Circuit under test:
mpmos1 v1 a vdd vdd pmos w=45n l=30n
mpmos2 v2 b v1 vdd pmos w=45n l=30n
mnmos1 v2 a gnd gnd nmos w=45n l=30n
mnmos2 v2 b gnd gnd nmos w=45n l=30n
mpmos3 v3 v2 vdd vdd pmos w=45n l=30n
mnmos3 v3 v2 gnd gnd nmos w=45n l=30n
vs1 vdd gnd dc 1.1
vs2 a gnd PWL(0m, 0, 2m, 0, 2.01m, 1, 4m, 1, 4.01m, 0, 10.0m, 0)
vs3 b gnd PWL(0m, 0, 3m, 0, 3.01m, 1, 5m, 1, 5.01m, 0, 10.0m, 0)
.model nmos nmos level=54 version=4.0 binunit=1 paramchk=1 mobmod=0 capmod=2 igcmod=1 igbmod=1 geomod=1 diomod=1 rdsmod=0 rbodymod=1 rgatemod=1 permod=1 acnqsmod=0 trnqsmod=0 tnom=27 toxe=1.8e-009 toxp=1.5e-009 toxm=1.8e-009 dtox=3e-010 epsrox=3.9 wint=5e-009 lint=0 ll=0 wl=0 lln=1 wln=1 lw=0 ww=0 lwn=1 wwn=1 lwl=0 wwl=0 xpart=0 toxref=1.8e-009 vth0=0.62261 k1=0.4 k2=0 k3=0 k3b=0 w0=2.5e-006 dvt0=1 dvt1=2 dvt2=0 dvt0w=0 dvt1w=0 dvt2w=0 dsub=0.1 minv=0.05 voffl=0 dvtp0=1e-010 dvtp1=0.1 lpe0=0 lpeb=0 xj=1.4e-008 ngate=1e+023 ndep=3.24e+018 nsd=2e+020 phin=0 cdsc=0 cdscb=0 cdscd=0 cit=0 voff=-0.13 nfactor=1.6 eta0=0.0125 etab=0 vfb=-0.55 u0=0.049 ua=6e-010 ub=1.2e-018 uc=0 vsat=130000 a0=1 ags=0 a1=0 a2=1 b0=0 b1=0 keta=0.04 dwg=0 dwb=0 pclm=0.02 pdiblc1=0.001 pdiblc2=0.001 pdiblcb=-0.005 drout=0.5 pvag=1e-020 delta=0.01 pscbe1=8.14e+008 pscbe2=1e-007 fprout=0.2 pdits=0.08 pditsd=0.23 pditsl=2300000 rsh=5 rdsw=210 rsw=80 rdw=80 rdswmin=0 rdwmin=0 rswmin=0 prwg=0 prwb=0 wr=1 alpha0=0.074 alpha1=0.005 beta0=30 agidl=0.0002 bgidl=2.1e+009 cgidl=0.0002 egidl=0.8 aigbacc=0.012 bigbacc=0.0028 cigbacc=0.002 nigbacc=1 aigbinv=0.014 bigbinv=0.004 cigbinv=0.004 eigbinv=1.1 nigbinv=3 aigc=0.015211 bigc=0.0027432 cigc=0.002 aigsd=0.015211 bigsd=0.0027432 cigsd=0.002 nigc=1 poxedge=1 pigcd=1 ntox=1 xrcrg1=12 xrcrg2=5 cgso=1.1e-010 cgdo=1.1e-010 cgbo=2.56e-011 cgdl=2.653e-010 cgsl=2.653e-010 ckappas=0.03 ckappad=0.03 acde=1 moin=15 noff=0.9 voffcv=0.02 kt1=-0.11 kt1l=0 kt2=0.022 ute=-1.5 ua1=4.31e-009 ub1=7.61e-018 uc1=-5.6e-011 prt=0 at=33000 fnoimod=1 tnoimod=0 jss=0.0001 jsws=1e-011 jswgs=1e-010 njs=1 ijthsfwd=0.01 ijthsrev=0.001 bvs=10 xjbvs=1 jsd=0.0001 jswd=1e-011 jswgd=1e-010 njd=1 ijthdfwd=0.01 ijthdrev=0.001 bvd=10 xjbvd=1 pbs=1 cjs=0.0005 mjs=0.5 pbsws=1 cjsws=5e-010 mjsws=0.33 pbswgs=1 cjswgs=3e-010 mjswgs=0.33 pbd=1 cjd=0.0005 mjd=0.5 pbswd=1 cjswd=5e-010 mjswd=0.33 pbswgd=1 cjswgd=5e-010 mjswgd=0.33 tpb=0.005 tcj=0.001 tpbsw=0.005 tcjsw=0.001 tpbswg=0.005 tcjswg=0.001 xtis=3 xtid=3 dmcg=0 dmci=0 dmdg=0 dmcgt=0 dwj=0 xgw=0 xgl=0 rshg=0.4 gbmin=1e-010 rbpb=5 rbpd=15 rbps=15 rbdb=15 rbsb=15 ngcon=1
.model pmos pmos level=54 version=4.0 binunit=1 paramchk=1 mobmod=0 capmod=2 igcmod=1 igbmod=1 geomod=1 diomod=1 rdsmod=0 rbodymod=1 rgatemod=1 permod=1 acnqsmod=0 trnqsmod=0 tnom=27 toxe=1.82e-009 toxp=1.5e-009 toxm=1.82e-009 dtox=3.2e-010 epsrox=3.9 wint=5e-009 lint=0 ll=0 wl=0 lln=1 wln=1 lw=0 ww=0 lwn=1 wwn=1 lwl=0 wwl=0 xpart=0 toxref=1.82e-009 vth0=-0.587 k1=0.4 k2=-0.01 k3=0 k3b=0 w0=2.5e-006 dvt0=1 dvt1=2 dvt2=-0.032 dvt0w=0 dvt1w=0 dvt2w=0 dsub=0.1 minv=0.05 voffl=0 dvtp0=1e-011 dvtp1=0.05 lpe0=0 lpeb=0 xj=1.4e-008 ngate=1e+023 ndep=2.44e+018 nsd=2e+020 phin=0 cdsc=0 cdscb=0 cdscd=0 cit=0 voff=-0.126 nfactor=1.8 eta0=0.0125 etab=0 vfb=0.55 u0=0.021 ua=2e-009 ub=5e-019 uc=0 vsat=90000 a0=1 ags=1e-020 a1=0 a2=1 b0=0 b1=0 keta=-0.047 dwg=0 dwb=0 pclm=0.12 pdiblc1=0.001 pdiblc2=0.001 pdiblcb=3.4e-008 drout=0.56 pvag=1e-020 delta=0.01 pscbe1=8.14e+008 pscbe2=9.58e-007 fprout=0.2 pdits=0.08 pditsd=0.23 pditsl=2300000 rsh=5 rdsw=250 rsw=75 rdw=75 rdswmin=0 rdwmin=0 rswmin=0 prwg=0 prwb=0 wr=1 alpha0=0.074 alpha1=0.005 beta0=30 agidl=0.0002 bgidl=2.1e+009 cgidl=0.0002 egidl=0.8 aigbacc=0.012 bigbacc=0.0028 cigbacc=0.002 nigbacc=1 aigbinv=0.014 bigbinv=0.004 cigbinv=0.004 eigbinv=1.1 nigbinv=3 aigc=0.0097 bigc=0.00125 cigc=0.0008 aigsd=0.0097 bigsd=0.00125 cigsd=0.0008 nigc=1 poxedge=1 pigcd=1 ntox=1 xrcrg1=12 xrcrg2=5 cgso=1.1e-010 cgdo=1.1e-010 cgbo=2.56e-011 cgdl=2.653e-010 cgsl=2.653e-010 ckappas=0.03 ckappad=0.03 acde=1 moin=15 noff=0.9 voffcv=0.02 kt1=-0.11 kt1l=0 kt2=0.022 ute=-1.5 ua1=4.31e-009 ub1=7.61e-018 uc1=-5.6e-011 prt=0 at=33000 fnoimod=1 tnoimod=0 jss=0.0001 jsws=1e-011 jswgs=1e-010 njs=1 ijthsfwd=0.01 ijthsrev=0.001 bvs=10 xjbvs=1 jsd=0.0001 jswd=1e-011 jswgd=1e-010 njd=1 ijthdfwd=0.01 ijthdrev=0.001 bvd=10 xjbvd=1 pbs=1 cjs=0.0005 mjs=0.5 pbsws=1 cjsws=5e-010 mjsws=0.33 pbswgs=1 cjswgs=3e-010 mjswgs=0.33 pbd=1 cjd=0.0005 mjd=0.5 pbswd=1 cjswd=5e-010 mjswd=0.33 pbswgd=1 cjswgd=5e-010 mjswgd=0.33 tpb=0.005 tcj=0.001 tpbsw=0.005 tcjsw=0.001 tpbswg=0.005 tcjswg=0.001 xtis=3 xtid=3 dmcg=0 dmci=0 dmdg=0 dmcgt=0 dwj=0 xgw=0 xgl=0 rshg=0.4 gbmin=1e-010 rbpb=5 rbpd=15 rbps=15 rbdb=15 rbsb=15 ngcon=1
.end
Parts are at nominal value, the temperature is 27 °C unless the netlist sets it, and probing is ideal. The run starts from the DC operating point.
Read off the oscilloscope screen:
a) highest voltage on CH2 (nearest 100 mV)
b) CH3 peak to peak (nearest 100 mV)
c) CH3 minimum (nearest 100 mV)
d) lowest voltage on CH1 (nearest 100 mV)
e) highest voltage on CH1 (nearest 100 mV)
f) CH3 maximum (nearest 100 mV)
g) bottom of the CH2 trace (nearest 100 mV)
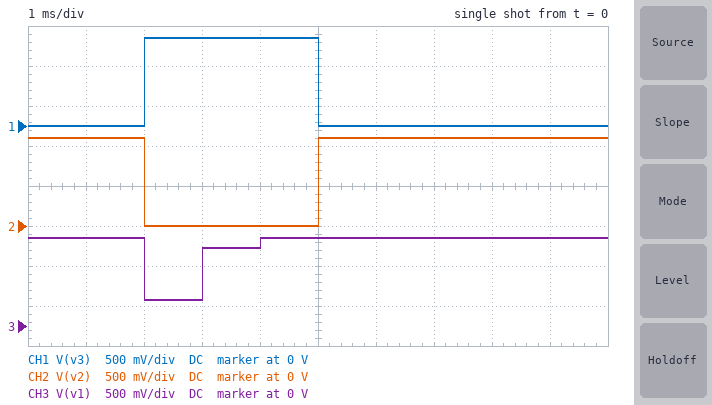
1.1 V
800 mV
300 mV
0 V
1.1 V
1.1 V
0 V
